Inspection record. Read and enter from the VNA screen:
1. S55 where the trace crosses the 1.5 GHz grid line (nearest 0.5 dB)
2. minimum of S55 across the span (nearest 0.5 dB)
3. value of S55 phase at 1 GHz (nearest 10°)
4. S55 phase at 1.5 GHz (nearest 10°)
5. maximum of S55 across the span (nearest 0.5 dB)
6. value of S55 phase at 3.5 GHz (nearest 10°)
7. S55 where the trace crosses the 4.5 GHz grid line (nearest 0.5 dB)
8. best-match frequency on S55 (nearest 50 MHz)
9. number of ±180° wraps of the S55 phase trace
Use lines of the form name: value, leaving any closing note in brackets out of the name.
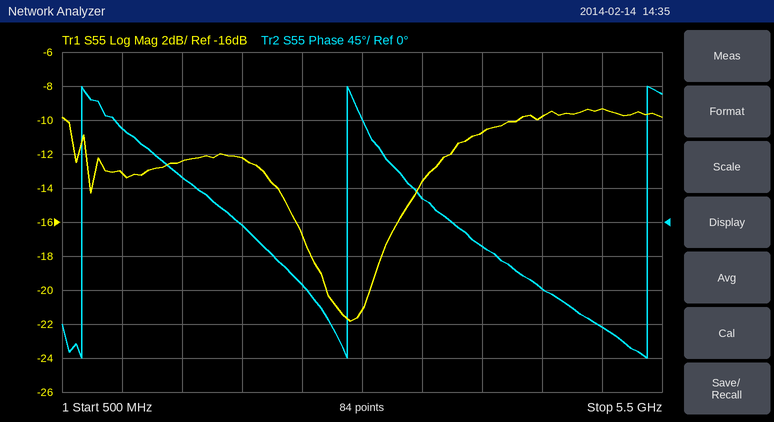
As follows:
S55 where the trace crosses the 1.5 GHz grid line: -12.5 dB
minimum of S55 across the span: -22.0 dB
value of S55 phase at 1 GHz: 120°
S55 phase at 1.5 GHz: 60°
maximum of S55 across the span: -9.5 dB
value of S55 phase at 3.5 GHz: 30°
S55 where the trace crosses the 4.5 GHz grid line: -10.0 dB
best-match frequency on S55: 2.90 GHz
number of ±180° wraps of the S55 phase trace: 3
